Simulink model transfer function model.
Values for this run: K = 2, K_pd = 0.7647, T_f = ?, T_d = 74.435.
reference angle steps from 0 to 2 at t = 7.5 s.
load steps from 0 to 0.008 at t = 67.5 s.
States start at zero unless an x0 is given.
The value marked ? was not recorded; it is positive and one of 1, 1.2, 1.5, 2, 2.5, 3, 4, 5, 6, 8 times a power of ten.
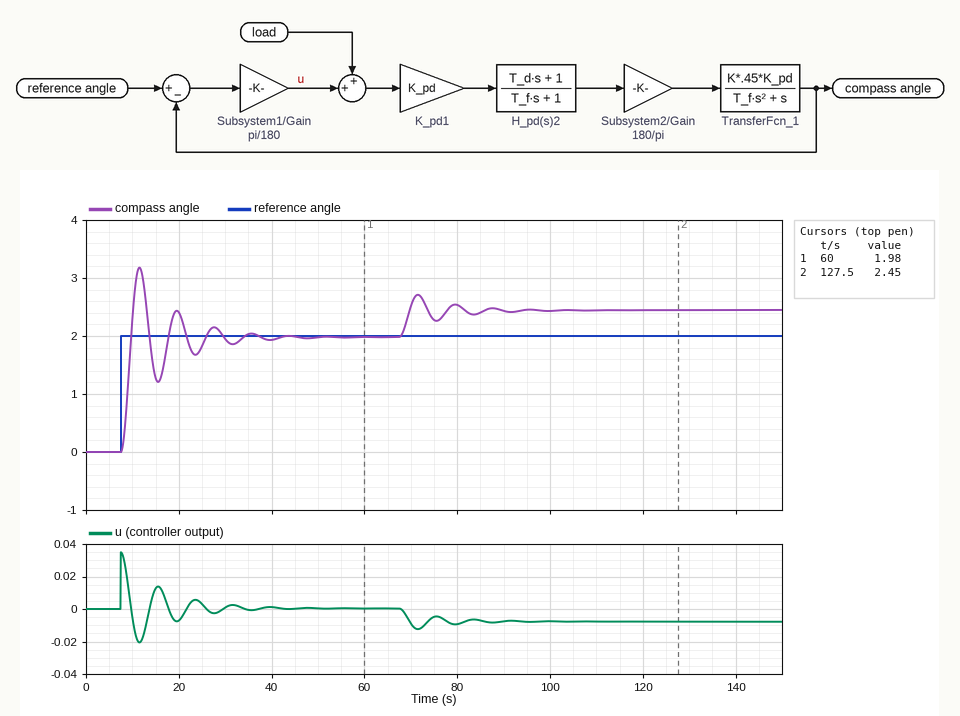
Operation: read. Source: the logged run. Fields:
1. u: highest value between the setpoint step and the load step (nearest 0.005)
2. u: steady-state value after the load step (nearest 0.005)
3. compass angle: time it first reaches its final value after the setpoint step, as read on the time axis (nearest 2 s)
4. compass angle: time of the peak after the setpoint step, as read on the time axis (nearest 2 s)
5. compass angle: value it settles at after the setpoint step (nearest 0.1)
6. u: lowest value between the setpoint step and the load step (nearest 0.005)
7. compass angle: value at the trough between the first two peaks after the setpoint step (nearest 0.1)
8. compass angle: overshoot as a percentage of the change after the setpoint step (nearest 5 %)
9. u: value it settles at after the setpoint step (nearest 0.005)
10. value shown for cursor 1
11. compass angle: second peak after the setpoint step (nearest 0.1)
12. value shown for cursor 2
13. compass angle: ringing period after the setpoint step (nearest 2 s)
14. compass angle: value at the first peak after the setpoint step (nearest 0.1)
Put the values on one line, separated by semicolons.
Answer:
0.035; -0.010; 10 s; 12 s; 2.0; -0.020; 1.2; 60 %; 0.000; 1.98; 2.4; 2.45; 8 s; 3.2
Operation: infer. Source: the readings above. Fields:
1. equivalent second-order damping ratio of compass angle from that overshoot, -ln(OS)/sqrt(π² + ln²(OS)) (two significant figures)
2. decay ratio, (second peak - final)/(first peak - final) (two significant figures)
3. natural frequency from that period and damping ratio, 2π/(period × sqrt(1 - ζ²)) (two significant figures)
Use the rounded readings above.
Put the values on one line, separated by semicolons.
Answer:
0.16; 0.33; 0.80 rad/s
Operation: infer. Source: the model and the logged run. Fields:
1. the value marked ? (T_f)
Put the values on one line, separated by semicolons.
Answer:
8
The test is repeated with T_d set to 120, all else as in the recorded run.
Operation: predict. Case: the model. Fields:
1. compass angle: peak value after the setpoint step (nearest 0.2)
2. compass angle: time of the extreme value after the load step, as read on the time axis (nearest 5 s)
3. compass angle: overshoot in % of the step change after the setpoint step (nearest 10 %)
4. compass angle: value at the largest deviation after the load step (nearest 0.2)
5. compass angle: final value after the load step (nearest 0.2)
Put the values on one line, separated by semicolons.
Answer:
3.4; 70 s; 70 %; 2.8; 2.4
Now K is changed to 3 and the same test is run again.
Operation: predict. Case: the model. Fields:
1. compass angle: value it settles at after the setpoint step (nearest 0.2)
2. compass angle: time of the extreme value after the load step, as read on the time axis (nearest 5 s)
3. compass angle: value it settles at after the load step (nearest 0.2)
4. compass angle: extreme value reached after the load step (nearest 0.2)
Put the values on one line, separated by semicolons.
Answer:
2.0; 70 s; 2.4; 2.8
